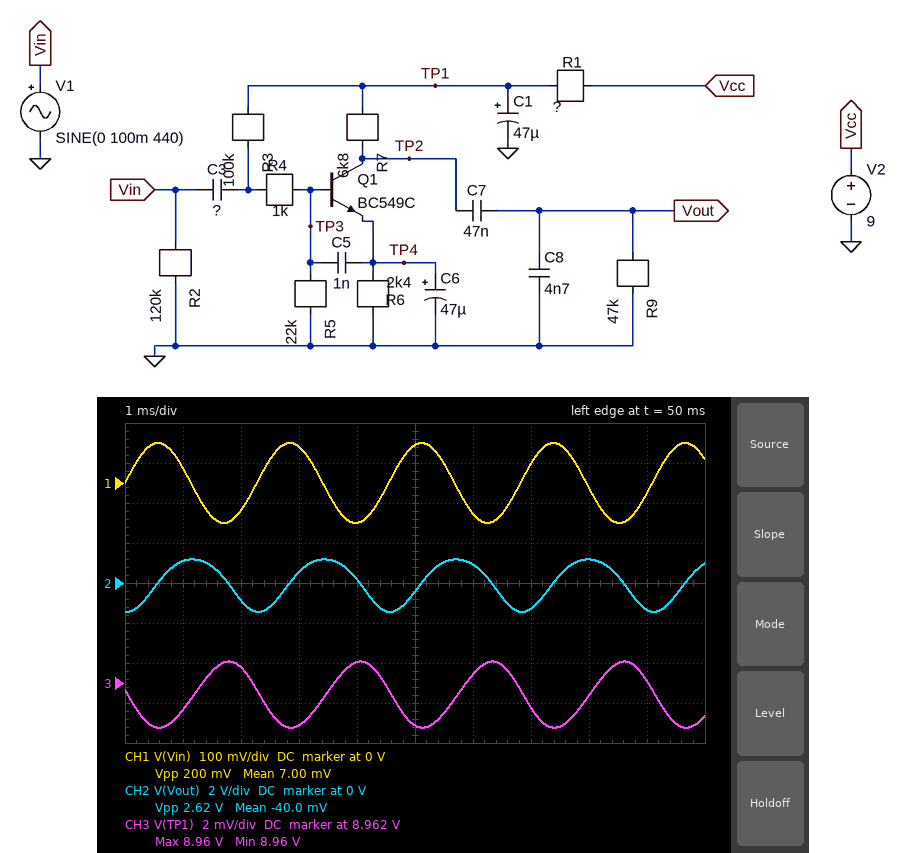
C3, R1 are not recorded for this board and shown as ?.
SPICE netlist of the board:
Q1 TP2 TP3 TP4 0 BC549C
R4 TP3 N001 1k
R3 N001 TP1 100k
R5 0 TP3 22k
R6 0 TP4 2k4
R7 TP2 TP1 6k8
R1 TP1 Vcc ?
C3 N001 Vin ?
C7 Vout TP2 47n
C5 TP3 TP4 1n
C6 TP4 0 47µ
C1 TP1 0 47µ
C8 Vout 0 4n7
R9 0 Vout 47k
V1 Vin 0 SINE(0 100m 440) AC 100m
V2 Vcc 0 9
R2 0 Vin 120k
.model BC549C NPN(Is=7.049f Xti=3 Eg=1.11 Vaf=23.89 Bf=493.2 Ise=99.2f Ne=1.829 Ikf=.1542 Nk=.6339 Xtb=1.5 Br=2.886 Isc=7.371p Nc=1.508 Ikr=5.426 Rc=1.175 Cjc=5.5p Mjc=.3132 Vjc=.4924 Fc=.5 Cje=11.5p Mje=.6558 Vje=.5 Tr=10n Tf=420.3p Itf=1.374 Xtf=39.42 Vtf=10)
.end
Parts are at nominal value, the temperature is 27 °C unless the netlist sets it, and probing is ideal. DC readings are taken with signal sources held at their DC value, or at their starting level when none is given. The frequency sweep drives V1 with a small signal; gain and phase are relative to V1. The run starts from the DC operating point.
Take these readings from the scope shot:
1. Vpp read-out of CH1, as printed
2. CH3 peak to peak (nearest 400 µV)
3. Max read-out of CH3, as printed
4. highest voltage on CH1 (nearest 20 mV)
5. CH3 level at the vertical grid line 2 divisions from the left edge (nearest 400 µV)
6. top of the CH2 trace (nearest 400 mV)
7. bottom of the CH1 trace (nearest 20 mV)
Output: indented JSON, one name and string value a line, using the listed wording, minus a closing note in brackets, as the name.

{
  "Vpp read-out of CH1, as printed": "200 mV",
  "CH3 peak to peak": "3.2 mV",
  "Max read-out of CH3, as printed": "8.96 V",
  "highest voltage on CH1": "100 mV",
  "CH3 level at the vertical grid line 2 divisions from the left edge": "8.9628 V",
  "top of the CH2 trace": "1.2 V",
  "bottom of the CH1 trace": "-100 mV"
}
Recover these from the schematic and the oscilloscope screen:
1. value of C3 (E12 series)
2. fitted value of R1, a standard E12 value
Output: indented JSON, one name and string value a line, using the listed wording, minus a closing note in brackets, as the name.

{
  "value of C3": "5.6 nF",
  "fitted value of R1, a standard E12 value": "82 Ω"
}
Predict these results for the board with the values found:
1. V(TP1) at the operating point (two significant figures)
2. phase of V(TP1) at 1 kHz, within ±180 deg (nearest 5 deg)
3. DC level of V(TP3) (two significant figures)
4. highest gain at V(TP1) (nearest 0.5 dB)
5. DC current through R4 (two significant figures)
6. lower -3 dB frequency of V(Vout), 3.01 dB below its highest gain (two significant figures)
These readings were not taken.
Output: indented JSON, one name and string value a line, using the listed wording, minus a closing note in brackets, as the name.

{
  "V(TP1) at the operating point": "9.0 V",
  "phase of V(TP1) at 1 kHz, within ±180 deg": "145 deg",
  "DC level of V(TP3)": "1.6 V",
  "highest gain at V(TP1)": "-35.0 dB",
  "DC current through R4": "73 µA",
  "lower -3 dB frequency of V(Vout), 3.01 dB below its highest gain": "1.3 kHz"
}
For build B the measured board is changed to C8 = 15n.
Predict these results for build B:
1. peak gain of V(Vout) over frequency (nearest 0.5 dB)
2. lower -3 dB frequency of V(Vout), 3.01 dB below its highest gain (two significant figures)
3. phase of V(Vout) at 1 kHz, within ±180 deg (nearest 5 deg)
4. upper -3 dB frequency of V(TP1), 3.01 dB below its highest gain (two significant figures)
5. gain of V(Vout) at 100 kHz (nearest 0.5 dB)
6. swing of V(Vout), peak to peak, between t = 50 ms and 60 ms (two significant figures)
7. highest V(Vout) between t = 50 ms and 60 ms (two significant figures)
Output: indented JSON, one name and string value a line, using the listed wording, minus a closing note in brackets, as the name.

{
  "peak gain of V(Vout) over frequency": "29.5 dB",
  "lower -3 dB frequency of V(Vout), 3.01 dB below its highest gain": "880 Hz",
  "phase of V(Vout) at 1 kHz, within ±180 deg": "-135 deg",
  "upper -3 dB frequency of V(TP1), 3.01 dB below its highest gain": "1.4 kHz",
  "gain of V(Vout) at 100 kHz": "1.0 dB",
  "swing of V(Vout), peak to peak, between t = 50 ms and 60 ms": "2.2 V",
  "highest V(Vout) between t = 50 ms and 60 ms": "1.0 V"
}
